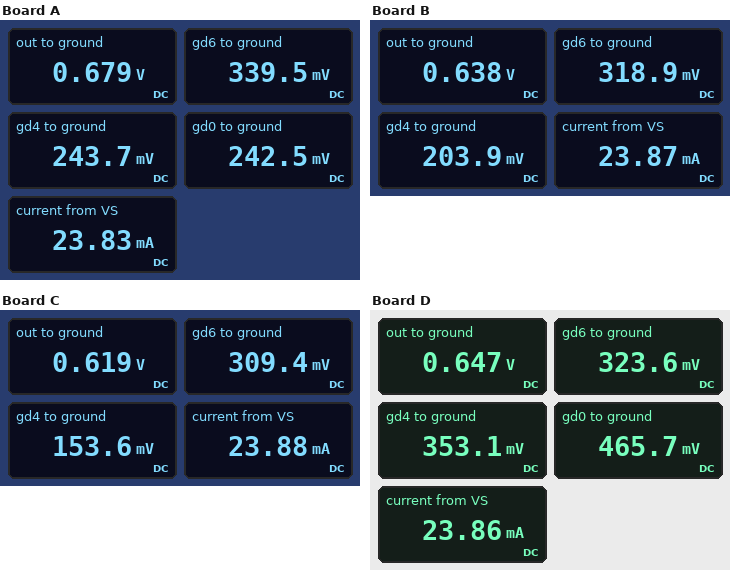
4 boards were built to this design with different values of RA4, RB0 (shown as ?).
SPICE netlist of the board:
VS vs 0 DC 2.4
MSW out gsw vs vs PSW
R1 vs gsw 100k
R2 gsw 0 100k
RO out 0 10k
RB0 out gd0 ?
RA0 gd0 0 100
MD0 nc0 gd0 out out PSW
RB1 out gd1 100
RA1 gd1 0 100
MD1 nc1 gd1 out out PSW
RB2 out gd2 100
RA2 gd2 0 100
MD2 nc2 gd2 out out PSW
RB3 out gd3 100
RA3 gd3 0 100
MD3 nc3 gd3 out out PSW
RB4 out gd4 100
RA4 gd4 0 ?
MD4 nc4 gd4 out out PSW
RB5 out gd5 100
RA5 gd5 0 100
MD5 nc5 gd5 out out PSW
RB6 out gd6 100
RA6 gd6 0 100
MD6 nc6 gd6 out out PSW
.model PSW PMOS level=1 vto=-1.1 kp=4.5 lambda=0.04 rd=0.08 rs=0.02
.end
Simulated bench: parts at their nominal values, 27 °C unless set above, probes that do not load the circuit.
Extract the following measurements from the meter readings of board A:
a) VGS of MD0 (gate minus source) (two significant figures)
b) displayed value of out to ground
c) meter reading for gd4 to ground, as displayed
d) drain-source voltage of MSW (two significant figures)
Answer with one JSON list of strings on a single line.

["-440 mV", "0.679 V", "243.7 mV", "-1.7 V"]
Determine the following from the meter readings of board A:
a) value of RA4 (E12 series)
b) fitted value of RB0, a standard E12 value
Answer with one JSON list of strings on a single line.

["56 Ω", "180 Ω"]
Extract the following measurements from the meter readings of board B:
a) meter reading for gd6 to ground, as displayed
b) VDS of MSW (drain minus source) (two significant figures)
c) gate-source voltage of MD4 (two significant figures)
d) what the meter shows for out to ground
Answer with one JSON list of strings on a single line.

["318.9 mV", "-1.8 V", "-430 mV", "0.638 V"]
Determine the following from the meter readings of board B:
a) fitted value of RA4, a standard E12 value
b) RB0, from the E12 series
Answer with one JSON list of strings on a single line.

["47 Ω", "82 Ω"]
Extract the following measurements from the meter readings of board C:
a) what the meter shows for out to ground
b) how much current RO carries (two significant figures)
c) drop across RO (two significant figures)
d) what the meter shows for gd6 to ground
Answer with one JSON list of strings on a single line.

["0.619 V", "62 µA", "620 mV", "309.4 mV"]
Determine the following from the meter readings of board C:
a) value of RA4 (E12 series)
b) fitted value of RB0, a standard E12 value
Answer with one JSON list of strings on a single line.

["33 Ω", "68 Ω"]
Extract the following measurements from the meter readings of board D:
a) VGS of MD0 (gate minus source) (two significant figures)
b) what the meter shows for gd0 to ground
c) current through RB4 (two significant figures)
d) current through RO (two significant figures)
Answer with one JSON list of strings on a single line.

["-180 mV", "465.7 mV", "2.9 mA", "65 µA"]
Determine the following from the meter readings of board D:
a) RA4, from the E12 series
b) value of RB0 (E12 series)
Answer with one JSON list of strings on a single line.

["120 Ω", "39 Ω"]
